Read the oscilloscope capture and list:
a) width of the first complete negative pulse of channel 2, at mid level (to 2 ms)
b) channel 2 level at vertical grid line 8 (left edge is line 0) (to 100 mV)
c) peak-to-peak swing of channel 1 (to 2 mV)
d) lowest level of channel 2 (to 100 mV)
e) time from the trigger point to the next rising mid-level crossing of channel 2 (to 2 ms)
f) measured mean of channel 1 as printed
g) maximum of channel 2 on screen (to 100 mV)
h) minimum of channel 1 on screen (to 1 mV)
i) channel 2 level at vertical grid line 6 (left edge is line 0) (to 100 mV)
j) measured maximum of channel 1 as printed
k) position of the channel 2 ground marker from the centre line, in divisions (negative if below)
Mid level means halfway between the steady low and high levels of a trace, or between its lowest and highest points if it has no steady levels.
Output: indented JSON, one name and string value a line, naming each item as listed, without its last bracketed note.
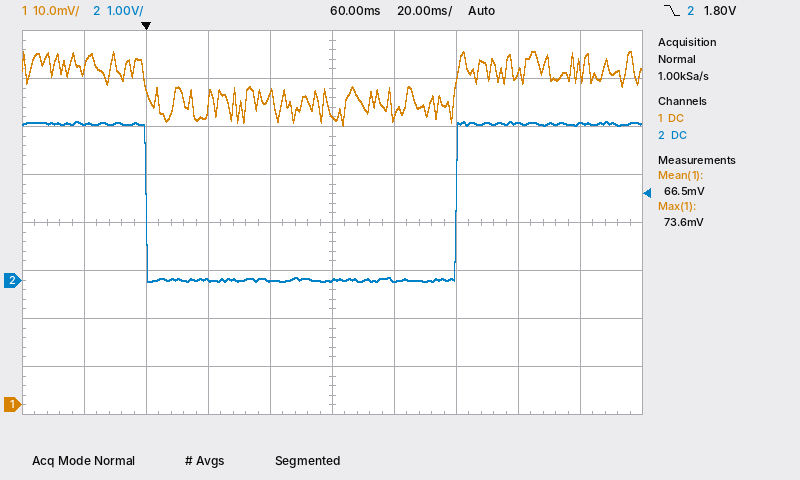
{
  "width of the first complete negative pulse of channel 2, at mid level": "100 ms",
  "channel 2 level at vertical grid line 8 (left edge is line 0)": "3.3 V",
  "peak-to-peak swing of channel 1": "16 mV",
  "lowest level of channel 2": "0.0 V",
  "time from the trigger point to the next rising mid-level crossing of channel 2": "100 ms",
  "measured mean of channel 1 as printed": "66.5 mV",
  "maximum of channel 2 on screen": "3.3 V",
  "minimum of channel 1 on screen": "58 mV",
  "channel 2 level at vertical grid line 6 (left edge is line 0)": "0.0 V",
  "measured maximum of channel 1 as printed": "73.6 mV",
  "position of the channel 2 ground marker from the centre line, in divisions": "-1.2 div"
}
